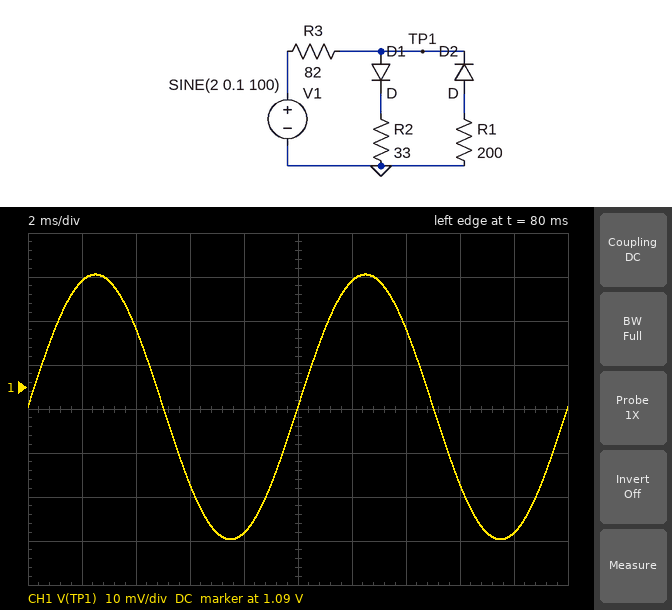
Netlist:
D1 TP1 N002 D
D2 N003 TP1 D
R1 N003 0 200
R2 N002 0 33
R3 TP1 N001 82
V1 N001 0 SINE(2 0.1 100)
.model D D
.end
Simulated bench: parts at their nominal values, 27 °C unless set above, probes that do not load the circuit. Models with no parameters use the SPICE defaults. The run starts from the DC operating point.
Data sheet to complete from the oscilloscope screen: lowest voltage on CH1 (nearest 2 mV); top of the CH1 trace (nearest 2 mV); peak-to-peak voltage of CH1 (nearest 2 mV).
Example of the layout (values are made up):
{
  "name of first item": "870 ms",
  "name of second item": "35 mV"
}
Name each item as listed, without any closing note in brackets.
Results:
{
  "lowest voltage on CH1": "1.056 V",
  "top of the CH1 trace": "1.116 V",
  "peak-to-peak voltage of CH1": "60 mV"
}
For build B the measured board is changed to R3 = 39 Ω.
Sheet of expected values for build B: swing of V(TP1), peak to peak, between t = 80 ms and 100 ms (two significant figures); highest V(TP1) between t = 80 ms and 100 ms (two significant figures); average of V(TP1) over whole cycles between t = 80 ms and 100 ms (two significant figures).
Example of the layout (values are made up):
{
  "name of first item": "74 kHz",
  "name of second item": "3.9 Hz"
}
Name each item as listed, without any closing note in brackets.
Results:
{
  "swing of V(TP1), peak to peak, between t = 80 ms and 100 ms": "94 mV",
  "highest V(TP1) between t = 80 ms and 100 ms": "1.4 V",
  "average of V(TP1) over whole cycles between t = 80 ms and 100 ms": "1.3 V"
}
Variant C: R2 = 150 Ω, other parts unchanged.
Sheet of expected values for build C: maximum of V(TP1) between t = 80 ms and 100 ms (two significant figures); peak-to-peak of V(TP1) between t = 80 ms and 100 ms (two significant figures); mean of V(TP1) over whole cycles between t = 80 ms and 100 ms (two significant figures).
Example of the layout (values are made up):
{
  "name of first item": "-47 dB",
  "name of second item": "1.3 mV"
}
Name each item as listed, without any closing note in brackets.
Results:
{
  "maximum of V(TP1) between t = 80 ms and 100 ms": "1.6 V",
  "peak-to-peak of V(TP1) between t = 80 ms and 100 ms": "130 mV",
  "mean of V(TP1) over whole cycles between t = 80 ms and 100 ms": "1.5 V"
}
